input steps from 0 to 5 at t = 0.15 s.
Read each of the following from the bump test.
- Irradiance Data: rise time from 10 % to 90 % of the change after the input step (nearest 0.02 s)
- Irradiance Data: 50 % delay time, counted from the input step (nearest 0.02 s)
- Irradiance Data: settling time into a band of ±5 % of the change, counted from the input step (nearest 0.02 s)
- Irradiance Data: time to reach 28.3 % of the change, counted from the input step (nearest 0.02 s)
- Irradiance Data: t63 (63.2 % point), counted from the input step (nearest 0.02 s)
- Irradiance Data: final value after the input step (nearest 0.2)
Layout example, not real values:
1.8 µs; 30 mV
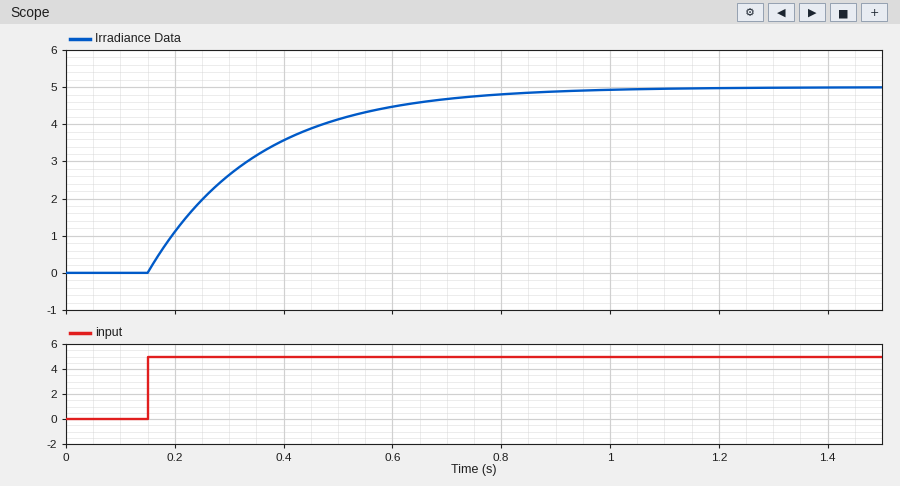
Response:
0.44 s; 0.14 s; 0.60 s; 0.06 s; 0.20 s; 5.0
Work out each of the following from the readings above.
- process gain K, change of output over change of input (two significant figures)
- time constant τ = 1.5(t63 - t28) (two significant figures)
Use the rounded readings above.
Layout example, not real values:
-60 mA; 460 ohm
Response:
1.0; 0.21 s
